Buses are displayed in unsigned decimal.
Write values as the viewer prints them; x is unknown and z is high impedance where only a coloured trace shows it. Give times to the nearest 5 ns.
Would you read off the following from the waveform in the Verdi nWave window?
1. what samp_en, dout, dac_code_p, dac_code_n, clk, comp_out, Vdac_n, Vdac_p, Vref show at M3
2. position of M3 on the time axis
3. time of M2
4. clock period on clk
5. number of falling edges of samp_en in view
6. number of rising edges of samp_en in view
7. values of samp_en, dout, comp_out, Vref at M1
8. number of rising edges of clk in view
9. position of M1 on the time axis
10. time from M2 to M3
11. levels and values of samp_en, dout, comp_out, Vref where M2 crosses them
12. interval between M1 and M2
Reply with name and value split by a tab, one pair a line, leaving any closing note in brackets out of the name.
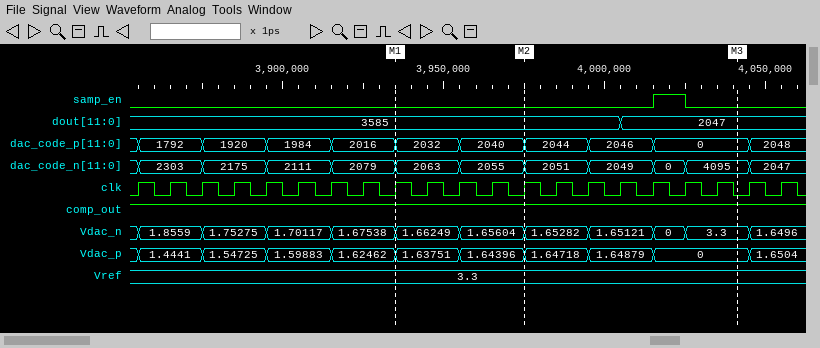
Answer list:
what samp_en, dout, dac_code_p, dac_code_n, clk, comp_out, Vdac_n, Vdac_p, Vref show at M3	samp_en=0, dout=2047, dac_code_p=0, dac_code_n=4095, clk=0, comp_out=1, Vdac_n=3.3, Vdac_p=0, Vref=3.3
position of M3 on the time axis	4040 ns
time of M2	3975 ns
clock period on clk	10 ns
number of falling edges of samp_en in view	1
number of rising edges of samp_en in view	1
values of samp_en, dout, comp_out, Vref at M1	samp_en=0, dout=3585, comp_out=1, Vref=3.3
number of rising edges of clk in view	21
position of M1 on the time axis	3935 ns
time from M2 to M3	65 ns
levels and values of samp_en, dout, comp_out, Vref where M2 crosses them	samp_en=0, dout=3585, comp_out=1, Vref=3.3
interval between M1 and M2	40 ns
